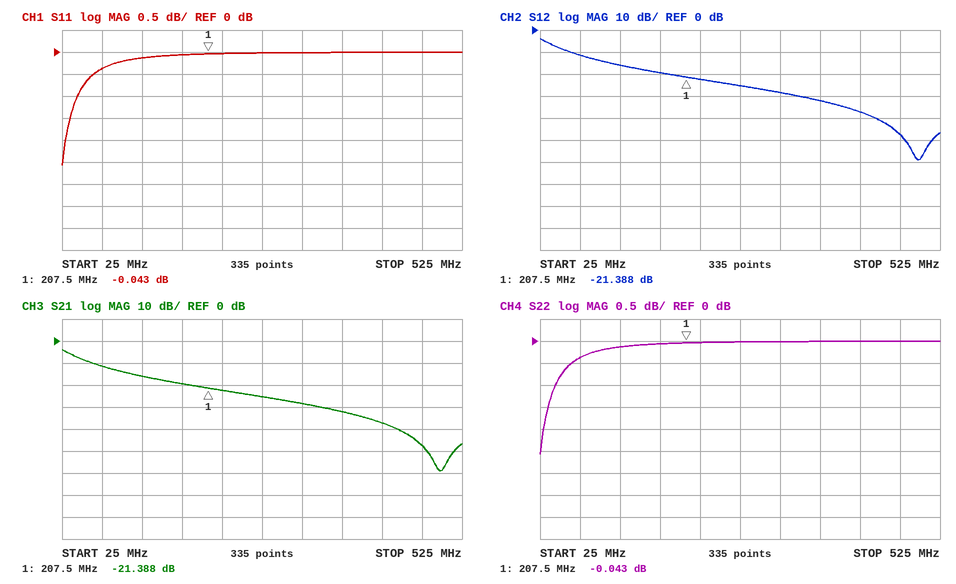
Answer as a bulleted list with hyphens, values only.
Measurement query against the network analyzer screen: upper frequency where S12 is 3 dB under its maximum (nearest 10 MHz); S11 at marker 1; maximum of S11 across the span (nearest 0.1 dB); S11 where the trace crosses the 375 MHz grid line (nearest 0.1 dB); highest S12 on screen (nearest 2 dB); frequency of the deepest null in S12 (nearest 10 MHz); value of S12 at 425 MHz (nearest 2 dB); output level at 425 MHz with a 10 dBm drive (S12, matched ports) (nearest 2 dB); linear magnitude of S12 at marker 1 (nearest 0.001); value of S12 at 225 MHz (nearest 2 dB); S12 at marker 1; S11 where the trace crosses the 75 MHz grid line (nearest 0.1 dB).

- 40 MHz
- -0.043 dB
- 0.0 dB
- 0.0 dB
- -4 dB
- 500 MHz
- -38 dB
- -28 dBm
- 0.085
- -22 dB
- -21.388 dB
- -0.4 dB
